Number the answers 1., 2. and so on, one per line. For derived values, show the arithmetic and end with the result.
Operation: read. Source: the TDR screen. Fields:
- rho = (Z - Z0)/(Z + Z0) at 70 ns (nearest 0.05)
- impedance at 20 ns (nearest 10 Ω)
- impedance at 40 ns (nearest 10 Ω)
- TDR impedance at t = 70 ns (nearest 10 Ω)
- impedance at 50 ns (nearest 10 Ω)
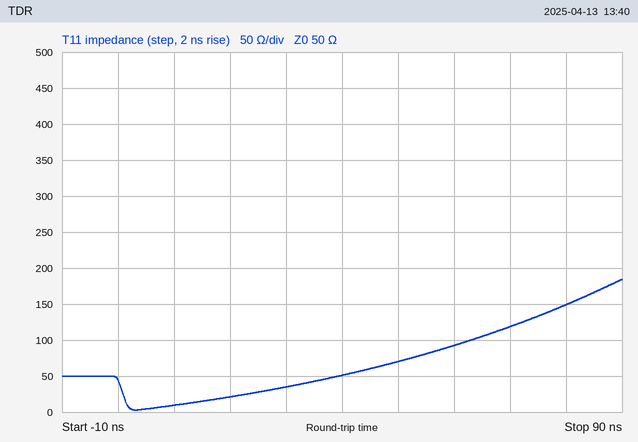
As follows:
1. (120 − 50)/(120 + 50) ≈ +0.412, so +0.40 to the nearest 0.05
2. 20 Ω
3. 50 Ω
4. 120 Ω
5. 70 Ω
